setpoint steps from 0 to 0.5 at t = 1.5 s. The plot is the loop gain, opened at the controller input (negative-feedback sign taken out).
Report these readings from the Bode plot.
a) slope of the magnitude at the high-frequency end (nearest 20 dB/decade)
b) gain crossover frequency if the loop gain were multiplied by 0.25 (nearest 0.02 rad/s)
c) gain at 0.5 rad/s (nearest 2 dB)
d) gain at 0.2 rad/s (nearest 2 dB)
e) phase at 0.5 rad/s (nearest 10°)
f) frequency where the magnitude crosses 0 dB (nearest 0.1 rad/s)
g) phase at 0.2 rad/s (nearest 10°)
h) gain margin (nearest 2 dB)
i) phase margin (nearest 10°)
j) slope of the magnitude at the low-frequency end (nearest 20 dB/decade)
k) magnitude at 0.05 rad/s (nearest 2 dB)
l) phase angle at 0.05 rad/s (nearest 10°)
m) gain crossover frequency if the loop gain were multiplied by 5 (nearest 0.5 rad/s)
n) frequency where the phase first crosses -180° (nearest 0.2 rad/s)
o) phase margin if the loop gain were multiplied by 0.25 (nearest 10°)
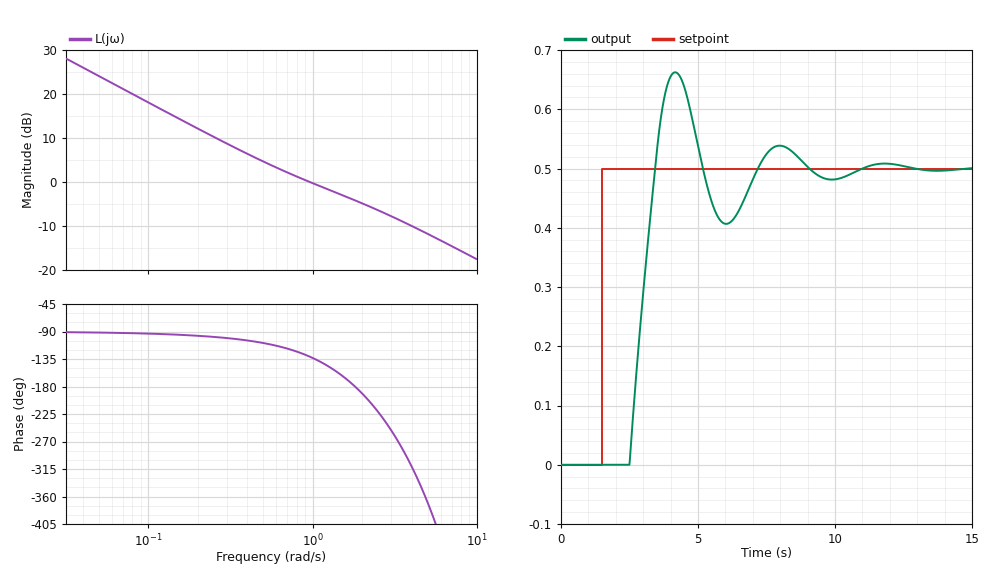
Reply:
-20 dB/decade
0.20 rad/s
4 dB
12 dB
-110°
1.0 rad/s
-100°
4 dB
50°
-20 dB/decade
24 dB
-90°
6.5 rad/s
1.8 rad/s
80°
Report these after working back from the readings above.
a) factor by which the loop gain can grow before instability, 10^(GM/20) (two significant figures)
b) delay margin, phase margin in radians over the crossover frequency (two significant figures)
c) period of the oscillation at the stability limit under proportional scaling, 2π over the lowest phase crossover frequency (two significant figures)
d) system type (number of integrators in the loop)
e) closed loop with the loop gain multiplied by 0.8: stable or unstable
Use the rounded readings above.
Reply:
1.6
0.87 s
3.5 s
1
stable
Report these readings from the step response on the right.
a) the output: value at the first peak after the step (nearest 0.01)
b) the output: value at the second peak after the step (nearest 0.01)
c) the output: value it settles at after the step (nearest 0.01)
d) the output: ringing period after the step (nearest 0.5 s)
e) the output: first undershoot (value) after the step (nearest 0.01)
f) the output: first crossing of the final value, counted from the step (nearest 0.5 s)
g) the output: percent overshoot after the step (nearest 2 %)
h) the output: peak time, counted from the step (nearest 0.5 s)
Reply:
0.66
0.54
0.50
4.0 s
0.41
2.0 s
32 %
2.5 s
